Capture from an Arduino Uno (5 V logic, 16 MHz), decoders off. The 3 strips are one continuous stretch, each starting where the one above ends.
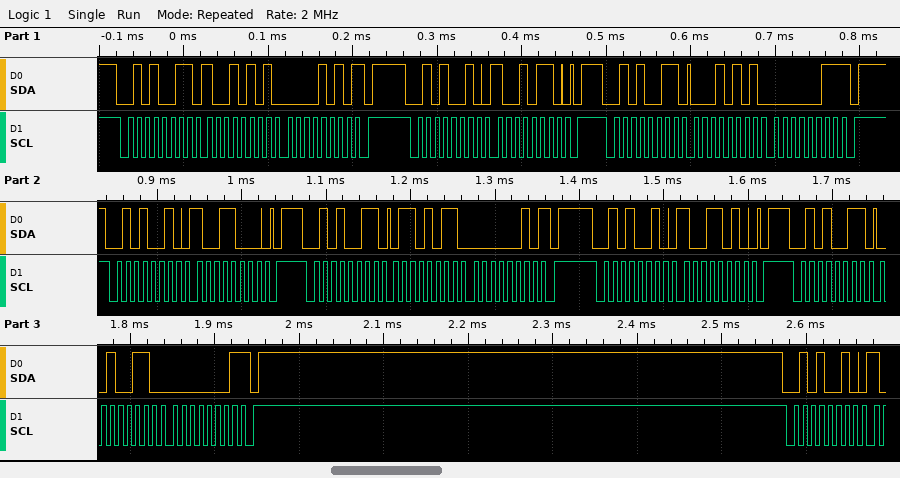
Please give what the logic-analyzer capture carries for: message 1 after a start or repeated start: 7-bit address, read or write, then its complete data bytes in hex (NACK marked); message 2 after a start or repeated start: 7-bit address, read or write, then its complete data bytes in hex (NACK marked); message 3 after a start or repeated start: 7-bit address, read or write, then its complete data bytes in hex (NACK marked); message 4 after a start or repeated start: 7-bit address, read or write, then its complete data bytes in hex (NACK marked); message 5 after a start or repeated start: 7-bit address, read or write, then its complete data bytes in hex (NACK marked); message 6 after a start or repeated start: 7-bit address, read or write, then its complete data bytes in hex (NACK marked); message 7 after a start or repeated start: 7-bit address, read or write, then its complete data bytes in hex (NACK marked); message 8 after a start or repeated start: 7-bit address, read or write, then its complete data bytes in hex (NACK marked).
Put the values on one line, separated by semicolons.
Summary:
0x29 read: 95 0A NACK; 0x29 write: 96; 0x29 read: 15 03 NACK; 0x29 write: 98; 0x29 read: 6B 02 NACK; 0x29 write: 9A; 0x29 read: 26 01 NACK; 0x29 write
